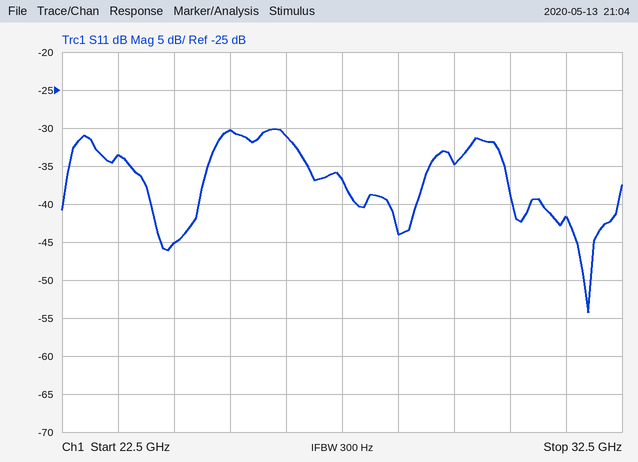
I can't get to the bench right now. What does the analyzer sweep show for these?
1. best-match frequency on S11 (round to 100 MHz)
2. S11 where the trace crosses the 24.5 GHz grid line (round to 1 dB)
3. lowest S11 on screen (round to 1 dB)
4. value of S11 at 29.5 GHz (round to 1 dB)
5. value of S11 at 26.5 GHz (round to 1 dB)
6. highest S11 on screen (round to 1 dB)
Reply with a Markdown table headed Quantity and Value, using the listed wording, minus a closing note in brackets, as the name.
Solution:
| Quantity | Value |
|---|---|
| best-match frequency on S11 | 31.9 GHz |
| S11 where the trace crosses the 24.5 GHz grid line | -45 dB |
| lowest S11 on screen | -54 dB |
| value of S11 at 29.5 GHz | -35 dB |
| value of S11 at 26.5 GHz | -31 dB |
| highest S11 on screen | -30 dB |
